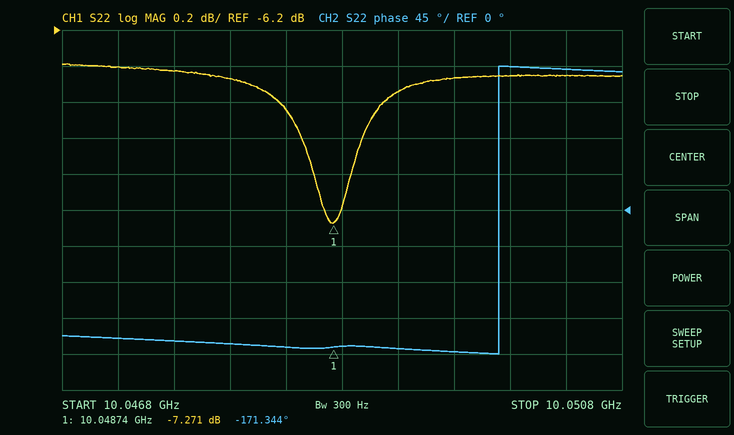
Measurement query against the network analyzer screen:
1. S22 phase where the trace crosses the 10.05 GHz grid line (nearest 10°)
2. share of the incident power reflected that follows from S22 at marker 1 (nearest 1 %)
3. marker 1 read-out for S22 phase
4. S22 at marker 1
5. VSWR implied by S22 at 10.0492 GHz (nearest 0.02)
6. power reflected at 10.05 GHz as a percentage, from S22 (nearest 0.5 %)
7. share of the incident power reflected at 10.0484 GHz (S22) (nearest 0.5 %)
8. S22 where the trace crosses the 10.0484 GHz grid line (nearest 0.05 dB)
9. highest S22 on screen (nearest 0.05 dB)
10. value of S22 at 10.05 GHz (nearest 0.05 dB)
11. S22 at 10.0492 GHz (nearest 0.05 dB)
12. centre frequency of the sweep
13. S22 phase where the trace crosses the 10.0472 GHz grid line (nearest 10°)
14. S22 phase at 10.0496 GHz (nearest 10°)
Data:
180°
19 %
-171.344°
-7.271 dB
2.78
22.5 %
21.5 %
-6.65 dB
-6.40 dB
-6.45 dB
-6.55 dB
10.0488 GHz
-160°
-180°
